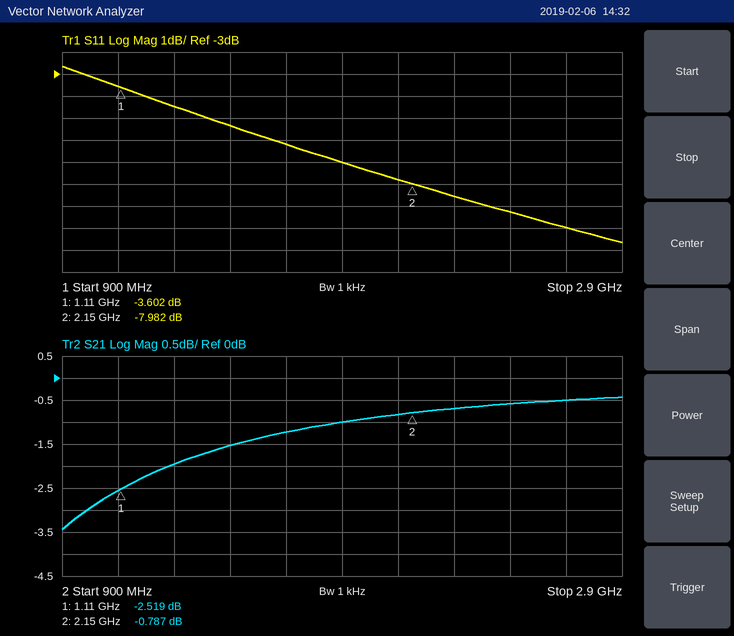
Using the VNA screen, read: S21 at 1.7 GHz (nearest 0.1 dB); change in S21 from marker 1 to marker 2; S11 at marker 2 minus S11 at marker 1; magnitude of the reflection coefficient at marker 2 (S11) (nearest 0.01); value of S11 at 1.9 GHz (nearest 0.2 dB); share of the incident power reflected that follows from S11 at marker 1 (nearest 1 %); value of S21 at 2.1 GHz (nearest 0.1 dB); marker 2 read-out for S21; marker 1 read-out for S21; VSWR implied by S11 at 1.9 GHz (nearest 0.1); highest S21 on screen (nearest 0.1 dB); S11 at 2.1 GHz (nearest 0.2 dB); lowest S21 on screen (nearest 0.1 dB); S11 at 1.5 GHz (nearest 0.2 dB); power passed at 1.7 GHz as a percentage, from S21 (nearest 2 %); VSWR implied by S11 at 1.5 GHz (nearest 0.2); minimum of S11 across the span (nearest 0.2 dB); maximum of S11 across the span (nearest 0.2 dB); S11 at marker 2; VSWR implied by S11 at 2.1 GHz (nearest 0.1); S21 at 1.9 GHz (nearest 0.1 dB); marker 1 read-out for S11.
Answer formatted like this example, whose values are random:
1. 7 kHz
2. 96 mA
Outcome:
1. -1.2 dB
2. 1.732 dB
3. -4.380 dB
4. 0.40
5. -7.0 dB
6. 44 %
7. -0.8 dB
8. -0.787 dB
9. -2.519 dB
10. 2.6
11. -0.4 dB
12. -7.8 dB
13. -3.4 dB
14. -5.4 dB
15. 76 %
16. 3.4
17. -10.6 dB
18. -2.6 dB
19. -7.982 dB
20. 2.4
21. -1.0 dB
22. -3.602 dB
